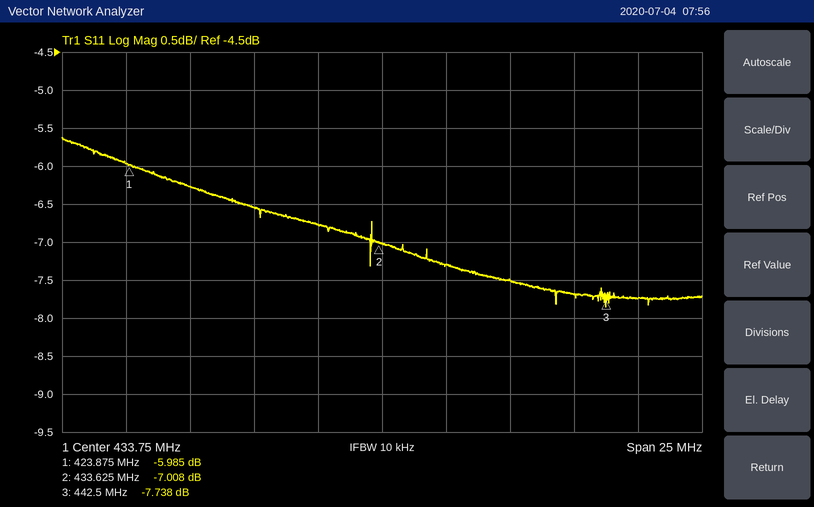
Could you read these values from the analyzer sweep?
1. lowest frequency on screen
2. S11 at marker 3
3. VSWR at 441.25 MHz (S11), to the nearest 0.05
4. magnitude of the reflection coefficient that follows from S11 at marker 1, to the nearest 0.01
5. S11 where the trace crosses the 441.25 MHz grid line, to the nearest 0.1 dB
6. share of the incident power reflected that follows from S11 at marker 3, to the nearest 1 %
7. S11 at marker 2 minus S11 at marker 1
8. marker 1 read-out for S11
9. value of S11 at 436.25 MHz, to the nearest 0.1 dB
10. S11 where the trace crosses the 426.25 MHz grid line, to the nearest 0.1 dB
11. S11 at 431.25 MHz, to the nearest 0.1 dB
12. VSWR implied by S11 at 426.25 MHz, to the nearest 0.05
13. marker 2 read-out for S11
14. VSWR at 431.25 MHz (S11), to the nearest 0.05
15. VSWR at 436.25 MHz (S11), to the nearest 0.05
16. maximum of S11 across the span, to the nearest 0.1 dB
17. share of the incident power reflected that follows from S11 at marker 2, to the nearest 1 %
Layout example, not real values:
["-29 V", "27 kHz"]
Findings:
["421.25 MHz", "-7.738 dB", "2.40", "0.50", "-7.7 dB", "17 %", "-1.023 dB", "-5.985 dB", "-7.3 dB", "-6.3 dB", "-6.8 dB", "2.90", "-7.008 dB", "2.70", "2.50", "-5.6 dB", "20 %"]
